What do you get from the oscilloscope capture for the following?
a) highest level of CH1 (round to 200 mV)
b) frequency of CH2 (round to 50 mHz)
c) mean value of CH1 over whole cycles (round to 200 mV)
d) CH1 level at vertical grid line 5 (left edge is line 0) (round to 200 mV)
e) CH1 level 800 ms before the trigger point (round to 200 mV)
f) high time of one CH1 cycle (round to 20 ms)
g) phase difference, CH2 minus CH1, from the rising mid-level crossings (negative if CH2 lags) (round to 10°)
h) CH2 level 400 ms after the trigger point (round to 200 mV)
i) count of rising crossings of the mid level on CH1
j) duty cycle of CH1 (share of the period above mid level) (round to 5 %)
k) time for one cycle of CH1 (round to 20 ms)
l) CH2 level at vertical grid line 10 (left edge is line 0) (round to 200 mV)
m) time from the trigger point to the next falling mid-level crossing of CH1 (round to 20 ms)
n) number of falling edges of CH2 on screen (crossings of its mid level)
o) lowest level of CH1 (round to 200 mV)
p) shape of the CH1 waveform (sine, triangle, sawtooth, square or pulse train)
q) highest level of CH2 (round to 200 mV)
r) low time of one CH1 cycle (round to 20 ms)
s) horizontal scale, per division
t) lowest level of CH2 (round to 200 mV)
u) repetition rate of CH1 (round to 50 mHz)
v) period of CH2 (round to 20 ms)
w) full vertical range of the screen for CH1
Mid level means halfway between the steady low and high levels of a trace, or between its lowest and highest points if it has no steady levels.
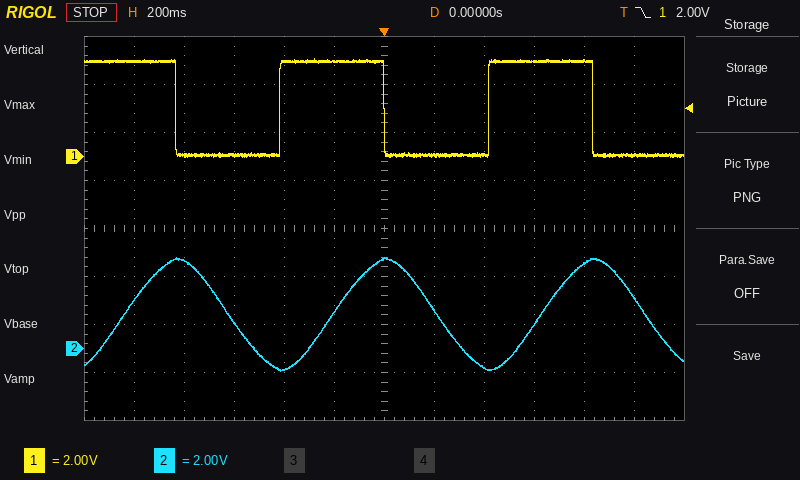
4.0 V
1.20 Hz
2.0 V
4.0 V
0.0 V
420 ms
-90°
-800 mV
2
50 %
840 ms
3.6 V
840 ms
3
0.0 V
square
3.8 V
420 ms
200 ms
-1.0 V
1.20 Hz
840 ms
16 V
